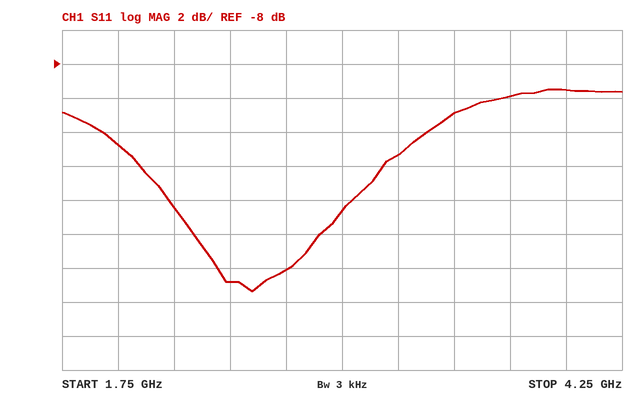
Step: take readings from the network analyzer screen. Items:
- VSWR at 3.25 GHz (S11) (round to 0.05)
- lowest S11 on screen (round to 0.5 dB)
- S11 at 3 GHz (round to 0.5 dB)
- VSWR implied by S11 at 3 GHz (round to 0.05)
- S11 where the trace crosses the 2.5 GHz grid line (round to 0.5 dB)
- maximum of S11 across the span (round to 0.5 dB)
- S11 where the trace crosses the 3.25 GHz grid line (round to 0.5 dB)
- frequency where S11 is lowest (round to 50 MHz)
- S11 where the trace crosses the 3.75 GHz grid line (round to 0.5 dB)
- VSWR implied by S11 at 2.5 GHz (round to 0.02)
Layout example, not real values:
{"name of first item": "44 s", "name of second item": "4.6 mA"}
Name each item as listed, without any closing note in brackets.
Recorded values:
{"VSWR at 3.25 GHz (S11)": "1.55", "lowest S11 on screen": "-21.5 dB", "S11 at 3 GHz": "-16.5 dB", "VSWR implied by S11 at 3 GHz": "1.35", "S11 where the trace crosses the 2.5 GHz grid line": "-21.0 dB", "maximum of S11 across the span": "-9.5 dB", "S11 where the trace crosses the 3.25 GHz grid line": "-13.5 dB", "frequency where S11 is lowest": "2.60 GHz", "S11 where the trace crosses the 3.75 GHz grid line": "-10.0 dB", "VSWR implied by S11 at 2.5 GHz": "1.20"}
